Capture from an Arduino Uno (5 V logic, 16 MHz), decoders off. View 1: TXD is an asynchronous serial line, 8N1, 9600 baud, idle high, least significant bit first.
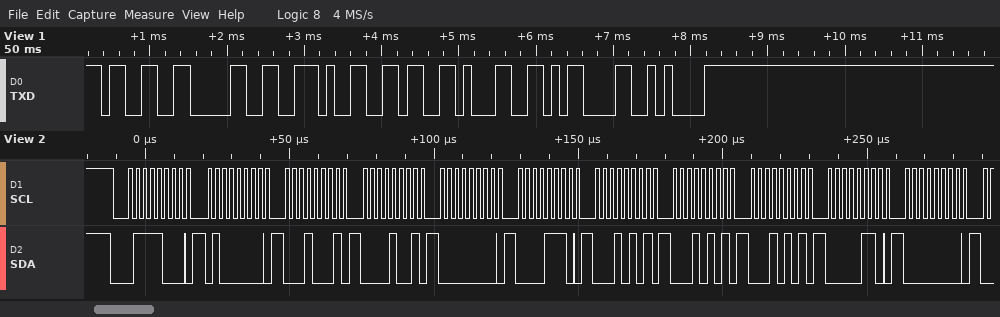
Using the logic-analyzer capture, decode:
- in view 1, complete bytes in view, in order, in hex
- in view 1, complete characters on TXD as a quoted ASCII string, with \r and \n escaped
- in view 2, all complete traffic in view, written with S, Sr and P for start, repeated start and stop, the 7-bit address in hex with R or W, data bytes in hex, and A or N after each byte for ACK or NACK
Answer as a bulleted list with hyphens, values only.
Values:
- 33 30 2E 36 31 0D 0A
- "30.61\r\n"
- S 3CW A 40 A 11 A 09 A 00 A 0E A 15 A 15 A 15 A 06 A 00 A
